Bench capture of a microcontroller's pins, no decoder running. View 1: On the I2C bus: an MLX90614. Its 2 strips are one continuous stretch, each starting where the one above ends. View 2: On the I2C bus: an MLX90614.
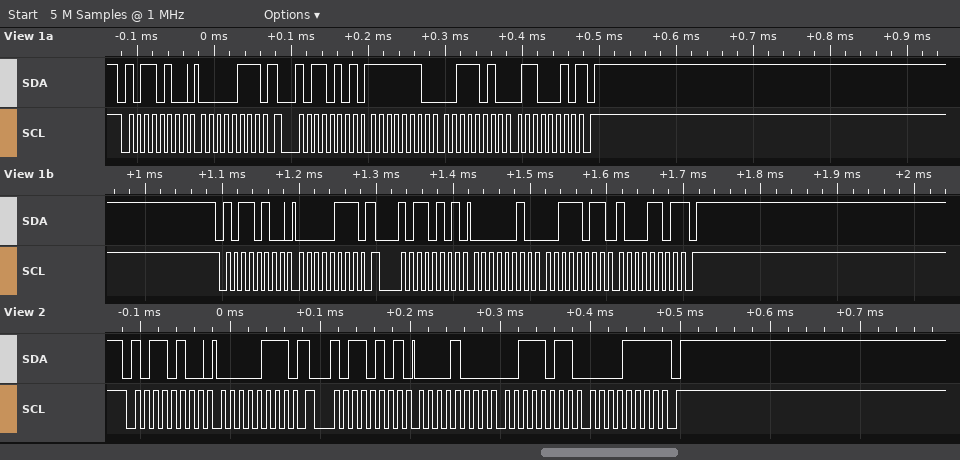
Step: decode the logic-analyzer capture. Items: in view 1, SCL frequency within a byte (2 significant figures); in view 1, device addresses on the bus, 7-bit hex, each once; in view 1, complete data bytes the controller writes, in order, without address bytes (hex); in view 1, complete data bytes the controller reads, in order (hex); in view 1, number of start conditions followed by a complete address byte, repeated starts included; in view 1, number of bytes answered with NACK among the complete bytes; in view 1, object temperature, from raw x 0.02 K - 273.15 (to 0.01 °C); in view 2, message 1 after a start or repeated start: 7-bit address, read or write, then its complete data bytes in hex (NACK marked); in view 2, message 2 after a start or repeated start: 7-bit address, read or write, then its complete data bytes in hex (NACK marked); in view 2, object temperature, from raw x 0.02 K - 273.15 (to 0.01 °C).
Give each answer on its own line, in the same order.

100 kHz
0x5A
07 07
FE 3A 62 02 3B 8D
4
2
28.89 °C
0x5A write: 07
0x5A read: 08 3B 0F NACK
29.09 °C
